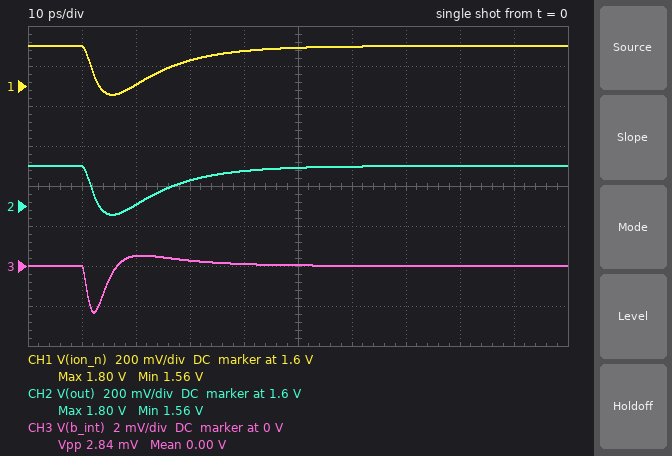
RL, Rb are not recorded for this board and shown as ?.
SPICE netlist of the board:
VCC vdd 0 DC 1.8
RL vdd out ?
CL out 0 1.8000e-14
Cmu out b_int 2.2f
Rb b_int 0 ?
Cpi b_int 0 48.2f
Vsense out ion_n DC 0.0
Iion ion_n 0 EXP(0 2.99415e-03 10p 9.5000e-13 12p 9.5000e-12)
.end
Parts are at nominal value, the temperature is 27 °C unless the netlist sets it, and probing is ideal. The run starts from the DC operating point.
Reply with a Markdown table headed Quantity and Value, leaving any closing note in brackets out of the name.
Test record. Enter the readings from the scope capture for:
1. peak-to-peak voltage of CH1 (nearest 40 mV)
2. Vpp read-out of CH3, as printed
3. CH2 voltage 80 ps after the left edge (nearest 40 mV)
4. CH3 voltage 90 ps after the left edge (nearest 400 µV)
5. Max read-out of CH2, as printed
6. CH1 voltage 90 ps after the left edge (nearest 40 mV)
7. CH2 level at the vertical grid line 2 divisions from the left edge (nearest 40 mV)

| Quantity | Value |
|---|---|
| peak-to-peak voltage of CH1 | 240 mV |
| Vpp read-out of CH3, as printed | 2.84 mV |
| CH2 voltage 80 ps after the left edge | 1.80 V |
| CH3 voltage 90 ps after the left edge | 0 V |
| Max read-out of CH2, as printed | 1.80 V |
| CH1 voltage 90 ps after the left edge | 1.80 V |
| CH2 level at the vertical grid line 2 divisions from the left edge | 1.60 V |
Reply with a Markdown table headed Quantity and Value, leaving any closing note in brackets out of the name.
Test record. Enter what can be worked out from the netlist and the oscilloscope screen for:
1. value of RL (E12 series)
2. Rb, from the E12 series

| Quantity | Value |
|---|---|
| value of RL | 120 Ω |
| Rb, from the E12 series | 15 Ω |
